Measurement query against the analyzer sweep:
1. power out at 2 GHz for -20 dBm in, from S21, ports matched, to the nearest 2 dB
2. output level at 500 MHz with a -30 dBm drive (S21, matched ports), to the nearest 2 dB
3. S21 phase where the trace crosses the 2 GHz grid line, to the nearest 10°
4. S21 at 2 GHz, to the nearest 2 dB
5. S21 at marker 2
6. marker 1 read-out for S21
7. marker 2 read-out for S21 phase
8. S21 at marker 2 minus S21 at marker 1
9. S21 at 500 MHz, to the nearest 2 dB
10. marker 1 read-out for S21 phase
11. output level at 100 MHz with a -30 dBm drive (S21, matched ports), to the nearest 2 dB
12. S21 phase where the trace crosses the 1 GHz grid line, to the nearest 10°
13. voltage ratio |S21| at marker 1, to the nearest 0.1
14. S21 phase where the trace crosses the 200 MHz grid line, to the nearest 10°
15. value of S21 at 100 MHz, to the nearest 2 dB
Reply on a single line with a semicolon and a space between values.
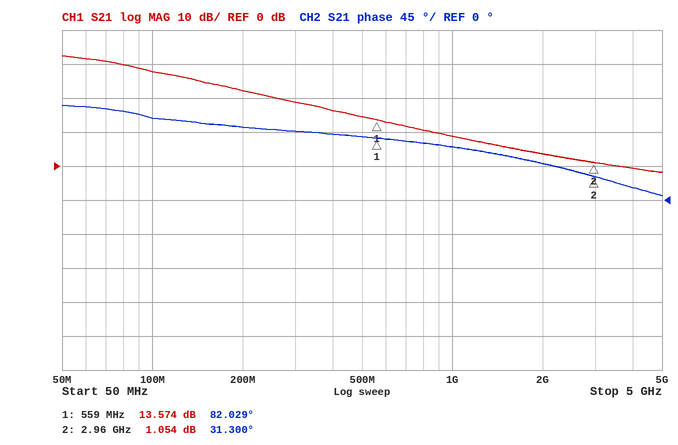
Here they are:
-16 dBm; -16 dBm; 50°; 4 dB; 1.054 dB; 13.574 dB; 31.300°; -12.520 dB; 14 dB; 82.029°; -2 dBm; 70°; 4.8; 100°; 28 dB
